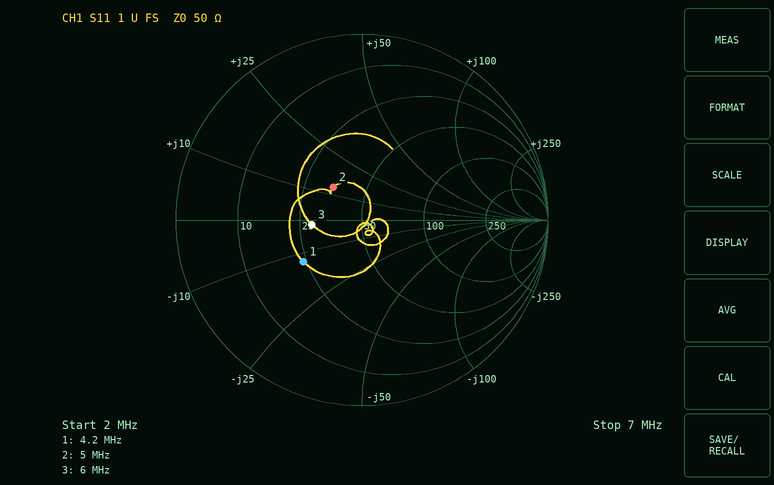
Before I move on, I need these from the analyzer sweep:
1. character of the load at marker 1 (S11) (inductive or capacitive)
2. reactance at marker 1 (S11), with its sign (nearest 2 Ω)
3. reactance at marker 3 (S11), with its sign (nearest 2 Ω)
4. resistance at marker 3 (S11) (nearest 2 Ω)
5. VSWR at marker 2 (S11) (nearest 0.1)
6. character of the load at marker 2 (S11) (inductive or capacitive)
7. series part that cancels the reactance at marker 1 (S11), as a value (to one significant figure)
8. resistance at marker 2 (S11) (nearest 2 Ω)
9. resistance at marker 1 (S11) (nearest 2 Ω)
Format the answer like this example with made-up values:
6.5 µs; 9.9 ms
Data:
capacitive; -12 Ω; -2 Ω; 28 Ω; 1.6; inductive; 500 nH; 34 Ω; 24 Ω
